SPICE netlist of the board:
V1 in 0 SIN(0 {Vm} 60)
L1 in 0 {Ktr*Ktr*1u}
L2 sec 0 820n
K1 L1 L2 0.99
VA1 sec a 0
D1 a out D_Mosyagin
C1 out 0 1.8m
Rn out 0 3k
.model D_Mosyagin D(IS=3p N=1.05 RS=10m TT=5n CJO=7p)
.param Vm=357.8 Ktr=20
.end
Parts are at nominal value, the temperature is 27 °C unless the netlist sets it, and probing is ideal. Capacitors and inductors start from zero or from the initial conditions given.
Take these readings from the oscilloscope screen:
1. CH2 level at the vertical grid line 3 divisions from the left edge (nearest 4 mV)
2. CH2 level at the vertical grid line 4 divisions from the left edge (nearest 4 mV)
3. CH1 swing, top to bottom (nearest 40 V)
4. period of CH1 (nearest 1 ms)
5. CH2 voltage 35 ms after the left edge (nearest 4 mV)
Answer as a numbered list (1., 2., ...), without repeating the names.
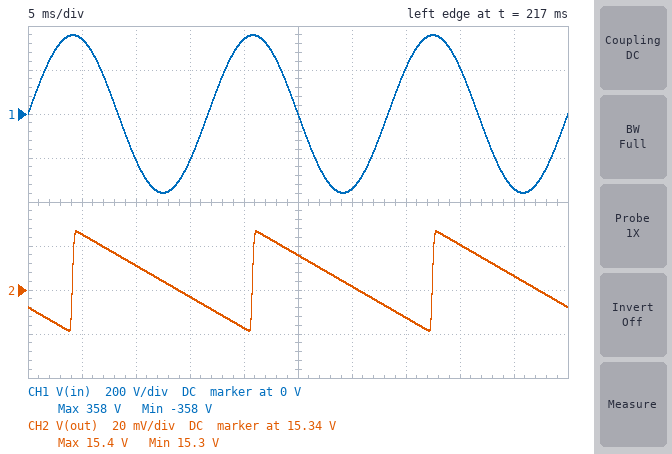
1. 15.336 V
2. 15.324 V
3. 720 V
4. 17 ms
5. 15.328 V
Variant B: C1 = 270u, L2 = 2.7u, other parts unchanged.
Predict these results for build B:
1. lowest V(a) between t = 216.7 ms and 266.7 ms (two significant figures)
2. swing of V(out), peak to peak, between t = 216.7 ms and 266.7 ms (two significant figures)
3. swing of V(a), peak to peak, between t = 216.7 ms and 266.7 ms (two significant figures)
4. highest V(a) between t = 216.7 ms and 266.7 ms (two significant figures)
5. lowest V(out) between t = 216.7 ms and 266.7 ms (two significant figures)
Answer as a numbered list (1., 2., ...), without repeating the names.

1. -29 V
2. 550 mV
3. 58 V
4. 29 V
5. 28 V
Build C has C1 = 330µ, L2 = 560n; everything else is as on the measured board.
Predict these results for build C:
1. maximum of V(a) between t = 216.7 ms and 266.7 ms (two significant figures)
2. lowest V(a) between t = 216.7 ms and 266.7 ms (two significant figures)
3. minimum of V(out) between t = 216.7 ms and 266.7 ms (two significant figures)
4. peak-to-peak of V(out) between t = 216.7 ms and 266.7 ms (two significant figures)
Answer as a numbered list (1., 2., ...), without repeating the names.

1. 13 V
2. -13 V
3. 12 V
4. 200 mV
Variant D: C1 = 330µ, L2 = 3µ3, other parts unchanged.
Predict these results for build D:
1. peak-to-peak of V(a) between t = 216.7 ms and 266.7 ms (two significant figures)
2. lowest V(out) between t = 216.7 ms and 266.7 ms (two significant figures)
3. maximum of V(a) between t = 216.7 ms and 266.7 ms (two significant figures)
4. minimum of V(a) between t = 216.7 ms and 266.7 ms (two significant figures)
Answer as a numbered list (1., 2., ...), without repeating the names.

1. 64 V
2. 31 V
3. 32 V
4. -32 V
